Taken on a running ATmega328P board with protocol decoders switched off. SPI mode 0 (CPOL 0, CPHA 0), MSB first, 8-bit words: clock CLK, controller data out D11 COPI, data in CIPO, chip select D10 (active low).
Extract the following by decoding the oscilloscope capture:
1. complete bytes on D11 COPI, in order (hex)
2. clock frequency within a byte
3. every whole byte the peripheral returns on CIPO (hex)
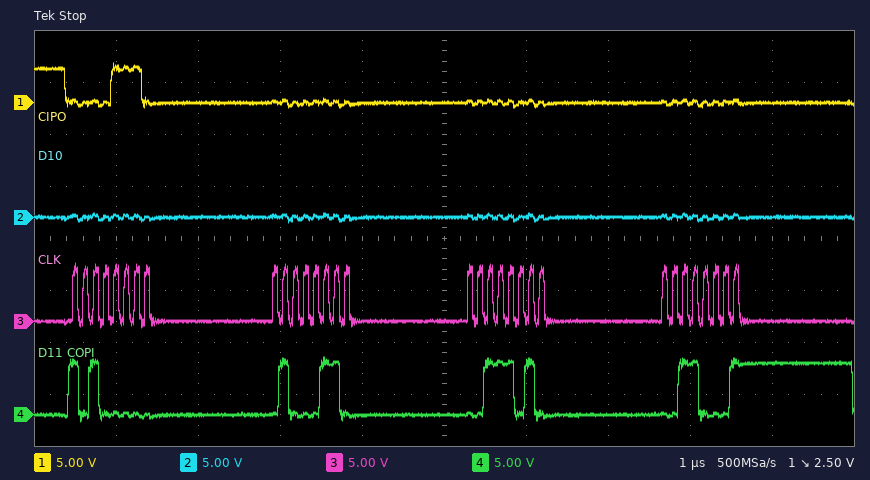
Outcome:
0xA0 0x46 0x3A 0x31
8 MHz
0x0E 0x00 0x00 0x00
